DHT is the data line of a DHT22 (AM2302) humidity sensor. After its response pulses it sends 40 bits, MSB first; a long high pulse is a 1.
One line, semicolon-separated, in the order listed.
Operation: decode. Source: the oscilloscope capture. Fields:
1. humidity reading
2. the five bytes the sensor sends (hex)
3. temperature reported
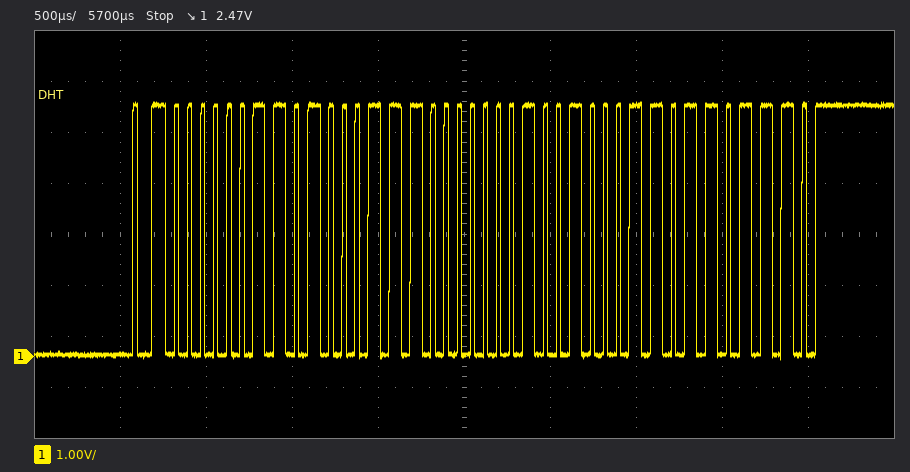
83.9 %; 03 47 01 23 6E; 29.1 °C
